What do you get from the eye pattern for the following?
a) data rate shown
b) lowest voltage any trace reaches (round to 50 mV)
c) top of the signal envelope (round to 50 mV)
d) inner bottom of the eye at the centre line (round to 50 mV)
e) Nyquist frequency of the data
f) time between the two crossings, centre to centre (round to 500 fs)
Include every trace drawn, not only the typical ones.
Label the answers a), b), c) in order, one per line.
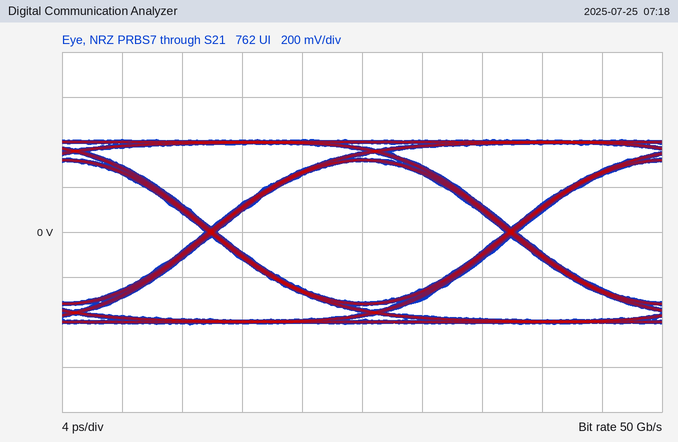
a) 50 Gb/s
b) -400 mV
c) 400 mV
d) -300 mV
e) 25 GHz
f) 20.0 ps
